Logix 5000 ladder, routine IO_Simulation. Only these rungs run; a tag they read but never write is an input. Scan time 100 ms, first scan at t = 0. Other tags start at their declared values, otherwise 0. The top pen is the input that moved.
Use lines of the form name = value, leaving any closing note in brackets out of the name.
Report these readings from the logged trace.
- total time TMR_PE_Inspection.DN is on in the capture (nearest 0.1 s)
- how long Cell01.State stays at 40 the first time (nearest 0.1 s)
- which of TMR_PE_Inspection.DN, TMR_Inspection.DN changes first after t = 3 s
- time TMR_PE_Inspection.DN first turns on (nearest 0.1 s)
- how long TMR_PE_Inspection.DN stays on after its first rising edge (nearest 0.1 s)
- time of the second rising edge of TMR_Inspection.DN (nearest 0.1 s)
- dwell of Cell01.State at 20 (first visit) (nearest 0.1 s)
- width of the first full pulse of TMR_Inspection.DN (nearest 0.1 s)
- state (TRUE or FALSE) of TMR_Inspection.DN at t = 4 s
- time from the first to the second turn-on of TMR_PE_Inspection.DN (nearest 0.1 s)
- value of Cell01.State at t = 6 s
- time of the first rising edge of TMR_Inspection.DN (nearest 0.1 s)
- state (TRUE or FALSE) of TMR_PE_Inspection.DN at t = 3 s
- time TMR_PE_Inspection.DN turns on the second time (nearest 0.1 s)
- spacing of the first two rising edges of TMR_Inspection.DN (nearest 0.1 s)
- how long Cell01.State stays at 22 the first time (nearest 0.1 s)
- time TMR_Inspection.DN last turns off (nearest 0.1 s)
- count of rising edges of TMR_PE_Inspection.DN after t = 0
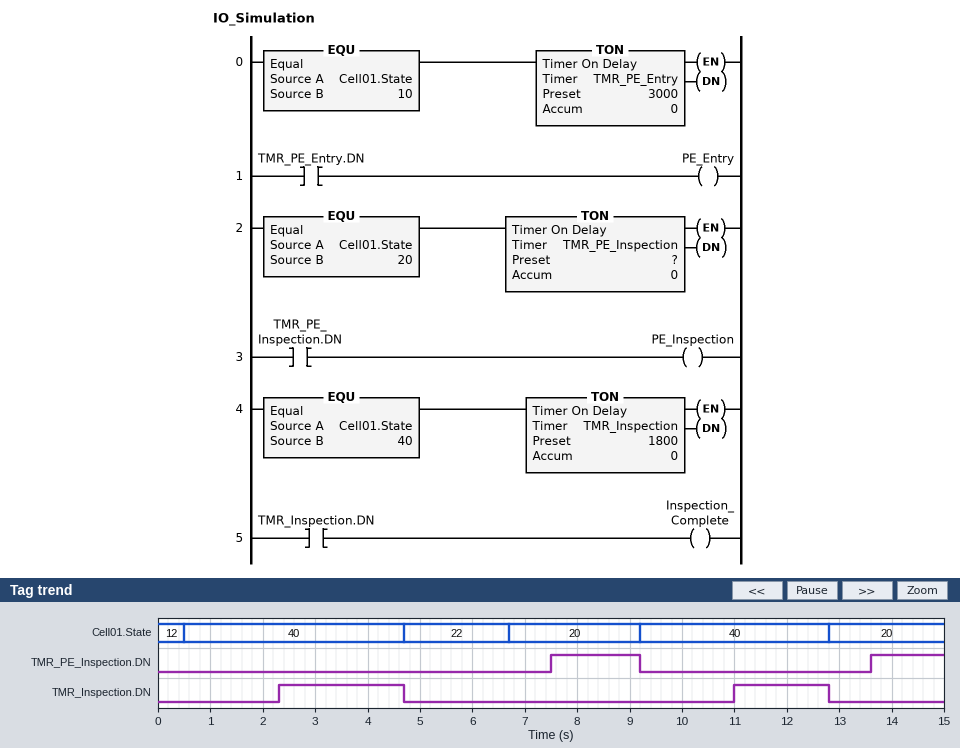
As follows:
total time TMR_PE_Inspection.DN is on in the capture = 3.1 s
how long Cell01.State stays at 40 the first time = 4.2 s
which of TMR_PE_Inspection.DN, TMR_Inspection.DN changes first after t = 3 s = TMR_Inspection.DN
time TMR_PE_Inspection.DN first turns on = 7.5 s
how long TMR_PE_Inspection.DN stays on after its first rising edge = 1.7 s
time of the second rising edge of TMR_Inspection.DN = 11.0 s
dwell of Cell01.State at 20 (first visit) = 2.5 s
width of the first full pulse of TMR_Inspection.DN = 2.4 s
state (TRUE or FALSE) of TMR_Inspection.DN at t = 4 s = TRUE
time from the first to the second turn-on of TMR_PE_Inspection.DN = 6.1 s
value of Cell01.State at t = 6 s = 22
time of the first rising edge of TMR_Inspection.DN = 2.3 s
state (TRUE or FALSE) of TMR_PE_Inspection.DN at t = 3 s = FALSE
time TMR_PE_Inspection.DN turns on the second time = 13.6 s
spacing of the first two rising edges of TMR_Inspection.DN = 8.7 s
how long Cell01.State stays at 22 the first time = 2.0 s
time TMR_Inspection.DN last turns off = 12.8 s
count of rising edges of TMR_PE_Inspection.DN after t = 0 = 2
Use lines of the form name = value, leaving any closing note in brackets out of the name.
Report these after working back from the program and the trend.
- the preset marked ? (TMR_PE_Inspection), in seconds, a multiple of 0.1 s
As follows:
the preset marked ? (TMR_PE_Inspection), in seconds, a multiple of 0.1 s = 0.8 s
